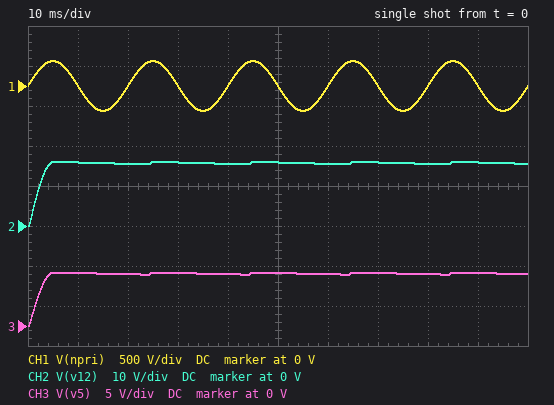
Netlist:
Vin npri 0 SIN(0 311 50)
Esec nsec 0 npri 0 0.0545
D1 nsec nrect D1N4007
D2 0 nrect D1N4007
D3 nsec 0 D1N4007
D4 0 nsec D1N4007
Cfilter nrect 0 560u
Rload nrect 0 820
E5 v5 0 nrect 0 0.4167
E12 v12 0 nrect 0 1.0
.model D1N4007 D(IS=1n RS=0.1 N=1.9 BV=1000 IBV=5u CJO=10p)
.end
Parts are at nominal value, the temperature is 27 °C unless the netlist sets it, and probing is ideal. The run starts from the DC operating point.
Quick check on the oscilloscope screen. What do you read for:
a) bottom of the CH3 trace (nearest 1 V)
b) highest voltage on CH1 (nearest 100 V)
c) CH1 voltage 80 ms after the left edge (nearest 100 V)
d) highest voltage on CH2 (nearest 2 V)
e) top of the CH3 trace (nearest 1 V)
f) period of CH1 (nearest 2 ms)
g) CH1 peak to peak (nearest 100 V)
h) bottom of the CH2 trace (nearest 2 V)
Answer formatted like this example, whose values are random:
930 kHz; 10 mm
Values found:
0 V; 300 V; 0 V; 16 V; 7 V; 20 ms; 600 V; 0 V
